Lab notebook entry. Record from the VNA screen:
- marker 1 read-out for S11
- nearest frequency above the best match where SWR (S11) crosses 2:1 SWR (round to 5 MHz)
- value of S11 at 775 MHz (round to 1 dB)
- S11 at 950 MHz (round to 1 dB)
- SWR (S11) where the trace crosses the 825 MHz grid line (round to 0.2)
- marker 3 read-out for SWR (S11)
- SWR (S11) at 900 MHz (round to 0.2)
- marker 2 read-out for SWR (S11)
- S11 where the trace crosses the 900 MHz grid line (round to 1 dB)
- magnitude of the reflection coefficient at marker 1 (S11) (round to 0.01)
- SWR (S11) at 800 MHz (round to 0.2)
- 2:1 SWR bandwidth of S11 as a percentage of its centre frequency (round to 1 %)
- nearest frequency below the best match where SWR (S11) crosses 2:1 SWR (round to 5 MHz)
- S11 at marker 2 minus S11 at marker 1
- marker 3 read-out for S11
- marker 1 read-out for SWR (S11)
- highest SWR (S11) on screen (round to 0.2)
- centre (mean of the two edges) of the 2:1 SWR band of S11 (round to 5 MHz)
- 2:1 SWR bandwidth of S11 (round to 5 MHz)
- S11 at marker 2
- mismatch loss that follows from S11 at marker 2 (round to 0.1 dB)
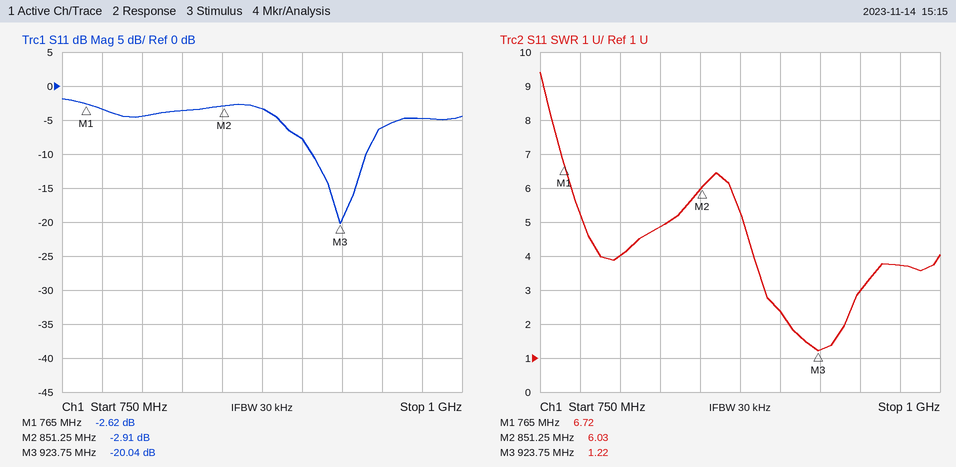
-2.62 dB
940 MHz
-3 dB
-6 dB
4.8
1.22
2.4
6.03
-8 dB
0.74
4.0
4 %
905 MHz
-0.29 dB
-20.04 dB
6.72
9.4
925 MHz
35 MHz
-2.91 dB
3.1 dB
